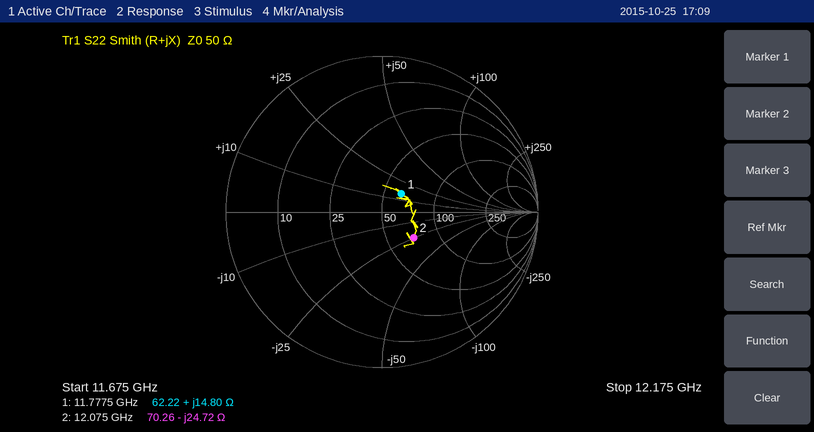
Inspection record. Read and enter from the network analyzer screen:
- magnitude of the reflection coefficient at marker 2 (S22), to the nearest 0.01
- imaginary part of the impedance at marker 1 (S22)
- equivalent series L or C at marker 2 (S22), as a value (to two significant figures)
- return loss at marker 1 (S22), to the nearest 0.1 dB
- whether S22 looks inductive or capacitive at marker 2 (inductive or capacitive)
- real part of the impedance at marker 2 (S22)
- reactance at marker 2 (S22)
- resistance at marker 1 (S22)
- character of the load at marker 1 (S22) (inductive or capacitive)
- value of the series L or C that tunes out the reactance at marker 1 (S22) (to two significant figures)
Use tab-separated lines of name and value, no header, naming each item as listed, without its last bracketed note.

magnitude of the reflection coefficient at marker 2 (S22), to the nearest 0.01	0.26
imaginary part of the impedance at marker 1	+14.80 Ω
equivalent series L or C at marker 2 (S22), as a value	530 fF
return loss at marker 1 (S22), to the nearest 0.1 dB	15.4 dB
whether S22 looks inductive or capacitive at marker 2	capacitive
real part of the impedance at marker 2	70.26 Ω
reactance at marker 2	-24.72 Ω
resistance at marker 1	62.22 Ω
character of the load at marker 1 (S22)	inductive
value of the series L or C that tunes out the reactance at marker 1 (S22)	910 fF
